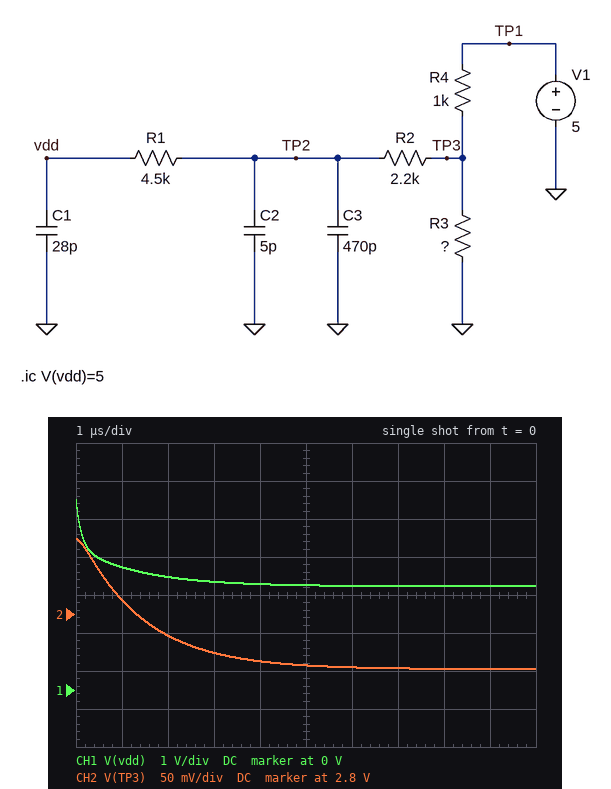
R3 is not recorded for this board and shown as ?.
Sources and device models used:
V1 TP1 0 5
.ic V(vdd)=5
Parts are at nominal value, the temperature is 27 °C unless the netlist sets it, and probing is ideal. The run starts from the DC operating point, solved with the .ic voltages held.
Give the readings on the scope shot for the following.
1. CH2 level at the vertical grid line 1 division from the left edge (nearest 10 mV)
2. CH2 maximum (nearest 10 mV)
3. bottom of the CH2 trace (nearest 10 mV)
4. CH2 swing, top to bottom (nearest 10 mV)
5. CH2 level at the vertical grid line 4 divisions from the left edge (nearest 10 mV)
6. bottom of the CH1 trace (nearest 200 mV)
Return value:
2.82 V
2.90 V
2.73 V
170 mV
2.74 V
2.8 V
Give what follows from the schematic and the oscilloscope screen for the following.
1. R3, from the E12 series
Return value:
1.2 kΩ
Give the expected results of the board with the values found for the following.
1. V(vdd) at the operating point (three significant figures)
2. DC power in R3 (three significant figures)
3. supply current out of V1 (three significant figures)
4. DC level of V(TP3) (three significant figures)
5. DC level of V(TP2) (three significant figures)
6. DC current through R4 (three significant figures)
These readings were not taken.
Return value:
2.73 V
6.20 mW
2.27 mA
2.73 V
2.73 V
2.27 mA
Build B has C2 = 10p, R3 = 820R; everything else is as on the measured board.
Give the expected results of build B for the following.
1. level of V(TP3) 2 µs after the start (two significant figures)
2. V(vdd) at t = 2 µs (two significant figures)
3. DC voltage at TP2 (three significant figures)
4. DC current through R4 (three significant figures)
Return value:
2.3 V
2.5 V
2.25 V
2.75 mA
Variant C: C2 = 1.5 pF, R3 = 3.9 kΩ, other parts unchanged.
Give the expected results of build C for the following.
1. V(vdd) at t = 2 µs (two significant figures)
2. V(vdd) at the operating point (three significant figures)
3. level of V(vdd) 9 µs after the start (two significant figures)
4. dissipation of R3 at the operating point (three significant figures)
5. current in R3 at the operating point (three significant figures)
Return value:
4.1 V
3.98 V
4.0 V
4.06 mW
1.02 mA
